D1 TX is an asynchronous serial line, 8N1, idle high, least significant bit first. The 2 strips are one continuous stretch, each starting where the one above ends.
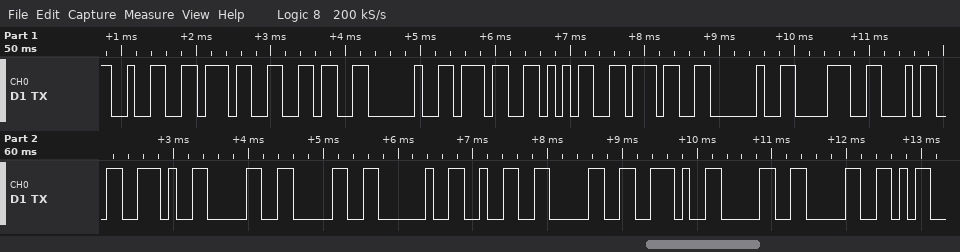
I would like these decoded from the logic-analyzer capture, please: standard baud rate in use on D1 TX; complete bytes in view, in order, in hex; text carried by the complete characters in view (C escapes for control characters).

9600 baud
32 37 36 20 37 35 37 20 38 34 2E 30 30 20 32 30 2E 30 30
"276 757 84.00 20.00"
